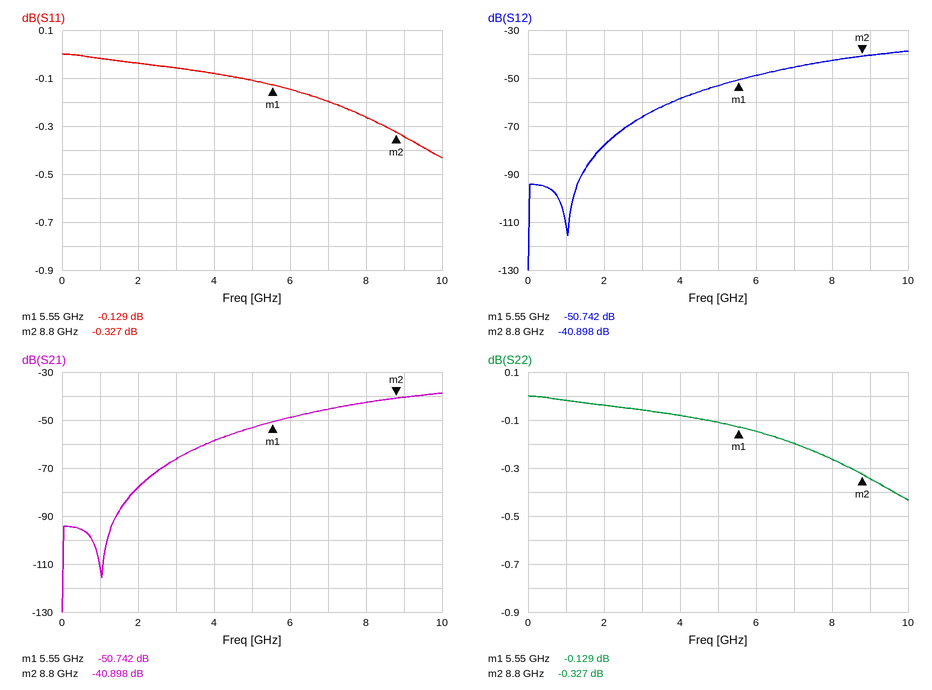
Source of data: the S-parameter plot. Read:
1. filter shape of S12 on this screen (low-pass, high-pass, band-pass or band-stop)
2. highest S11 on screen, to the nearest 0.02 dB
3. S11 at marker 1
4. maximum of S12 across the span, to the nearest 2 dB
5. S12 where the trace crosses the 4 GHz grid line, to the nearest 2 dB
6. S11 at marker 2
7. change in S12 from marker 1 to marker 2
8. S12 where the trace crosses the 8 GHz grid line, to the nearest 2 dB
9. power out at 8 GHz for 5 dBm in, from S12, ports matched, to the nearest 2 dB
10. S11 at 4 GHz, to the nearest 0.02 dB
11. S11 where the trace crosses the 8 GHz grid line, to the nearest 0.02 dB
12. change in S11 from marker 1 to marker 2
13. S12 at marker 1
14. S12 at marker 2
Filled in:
high-pass
0.00 dB
-0.129 dB
-38 dB
-58 dB
-0.327 dB
9.844 dB
-42 dB
-38 dBm
-0.08 dB
-0.26 dB
-0.198 dB
-50.742 dB
-40.898 dB
